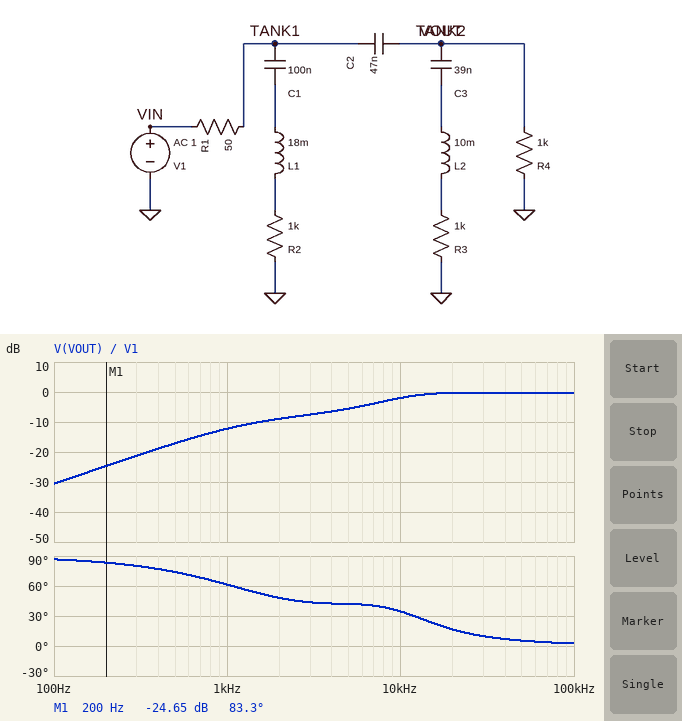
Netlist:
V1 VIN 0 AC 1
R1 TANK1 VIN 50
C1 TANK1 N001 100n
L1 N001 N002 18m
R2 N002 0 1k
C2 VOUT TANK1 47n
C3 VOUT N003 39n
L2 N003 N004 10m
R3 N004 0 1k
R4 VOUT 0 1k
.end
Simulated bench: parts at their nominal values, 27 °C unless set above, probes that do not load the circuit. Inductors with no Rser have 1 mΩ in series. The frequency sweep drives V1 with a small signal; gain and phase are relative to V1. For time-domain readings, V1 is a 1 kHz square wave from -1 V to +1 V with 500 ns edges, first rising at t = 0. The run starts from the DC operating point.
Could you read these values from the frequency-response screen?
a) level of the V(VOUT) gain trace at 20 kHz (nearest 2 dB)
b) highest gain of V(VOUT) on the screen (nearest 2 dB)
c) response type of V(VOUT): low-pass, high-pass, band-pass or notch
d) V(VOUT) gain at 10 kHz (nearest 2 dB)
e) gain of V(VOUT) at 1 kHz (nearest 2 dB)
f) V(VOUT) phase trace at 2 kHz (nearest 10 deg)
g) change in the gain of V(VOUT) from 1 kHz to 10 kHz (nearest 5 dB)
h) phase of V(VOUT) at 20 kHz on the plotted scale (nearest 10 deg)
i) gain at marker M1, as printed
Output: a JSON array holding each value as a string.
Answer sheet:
["0 dB", "0 dB", "high-pass", "-2 dB", "-12 dB", "50 deg", "10 dB", "20 deg", "-24.65 dB"]
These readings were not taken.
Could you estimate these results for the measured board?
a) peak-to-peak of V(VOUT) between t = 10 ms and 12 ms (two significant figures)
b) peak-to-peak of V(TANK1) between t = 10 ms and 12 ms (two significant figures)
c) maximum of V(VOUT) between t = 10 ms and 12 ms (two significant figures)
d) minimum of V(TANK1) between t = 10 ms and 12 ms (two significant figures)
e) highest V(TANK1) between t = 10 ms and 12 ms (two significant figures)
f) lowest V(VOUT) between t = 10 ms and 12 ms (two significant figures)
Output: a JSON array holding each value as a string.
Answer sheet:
["3.8 V", "2.0 V", "1.9 V", "-1.0 V", "1.0 V", "-1.9 V"]
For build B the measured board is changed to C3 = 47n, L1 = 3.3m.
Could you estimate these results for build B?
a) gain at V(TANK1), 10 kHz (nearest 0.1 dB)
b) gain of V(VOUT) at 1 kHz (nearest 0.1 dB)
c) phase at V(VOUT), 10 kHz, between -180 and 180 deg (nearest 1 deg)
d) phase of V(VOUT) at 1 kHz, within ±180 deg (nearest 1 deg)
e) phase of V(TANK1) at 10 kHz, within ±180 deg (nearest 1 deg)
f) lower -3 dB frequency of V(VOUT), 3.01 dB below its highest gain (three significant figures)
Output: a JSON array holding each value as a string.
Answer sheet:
["-1.0 dB", "-12.5 dB", "34 deg", "60 deg", "-2 deg", "7.49 kHz"]
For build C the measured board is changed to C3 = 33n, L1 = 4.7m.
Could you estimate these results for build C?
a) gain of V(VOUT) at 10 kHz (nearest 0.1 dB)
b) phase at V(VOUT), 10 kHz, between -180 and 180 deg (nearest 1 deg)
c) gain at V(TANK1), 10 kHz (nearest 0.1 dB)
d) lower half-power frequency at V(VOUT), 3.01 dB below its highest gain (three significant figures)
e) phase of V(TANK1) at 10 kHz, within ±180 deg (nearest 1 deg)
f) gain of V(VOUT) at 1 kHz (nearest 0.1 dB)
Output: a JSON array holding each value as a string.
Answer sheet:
["-2.3 dB", "33 deg", "-1.0 dB", "7.98 kHz", "-2 deg", "-12.0 dB"]
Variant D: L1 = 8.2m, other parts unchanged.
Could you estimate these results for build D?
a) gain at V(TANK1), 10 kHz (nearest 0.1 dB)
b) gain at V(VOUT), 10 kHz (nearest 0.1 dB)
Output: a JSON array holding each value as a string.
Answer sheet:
["-1.0 dB", "-2.1 dB"]
